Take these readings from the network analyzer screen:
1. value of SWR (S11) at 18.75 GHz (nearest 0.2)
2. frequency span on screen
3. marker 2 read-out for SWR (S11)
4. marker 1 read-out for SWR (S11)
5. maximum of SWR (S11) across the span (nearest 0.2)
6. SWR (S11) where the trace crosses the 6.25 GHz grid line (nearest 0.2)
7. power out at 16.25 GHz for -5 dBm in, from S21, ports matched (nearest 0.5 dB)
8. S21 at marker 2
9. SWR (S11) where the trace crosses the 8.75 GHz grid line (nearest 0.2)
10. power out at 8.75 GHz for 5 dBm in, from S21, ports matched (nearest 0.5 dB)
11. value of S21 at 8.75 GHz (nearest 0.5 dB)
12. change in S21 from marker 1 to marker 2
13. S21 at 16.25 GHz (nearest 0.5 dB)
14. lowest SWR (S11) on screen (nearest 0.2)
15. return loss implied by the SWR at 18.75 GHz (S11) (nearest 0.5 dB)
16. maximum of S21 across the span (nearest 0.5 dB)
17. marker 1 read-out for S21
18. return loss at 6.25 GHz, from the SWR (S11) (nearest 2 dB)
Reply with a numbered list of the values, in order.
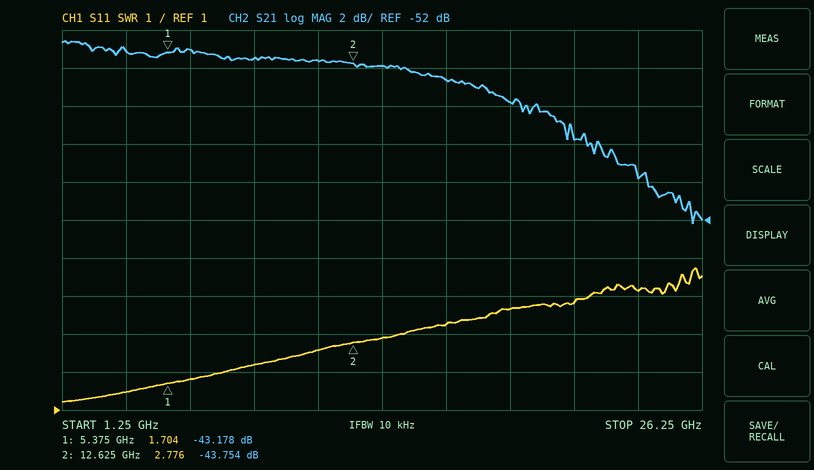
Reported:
1. 3.6
2. 25 GHz
3. 2.776
4. 1.704
5. 4.8
6. 1.8
7. -49.5 dBm
8. -43.754 dB
9. 2.2
10. -38.5 dBm
11. -43.5 dB
12. -0.576 dB
13. -44.5 dB
14. 1.2
15. 5.0 dB
16. -42.5 dB
17. -43.178 dB
18. 10 dB
